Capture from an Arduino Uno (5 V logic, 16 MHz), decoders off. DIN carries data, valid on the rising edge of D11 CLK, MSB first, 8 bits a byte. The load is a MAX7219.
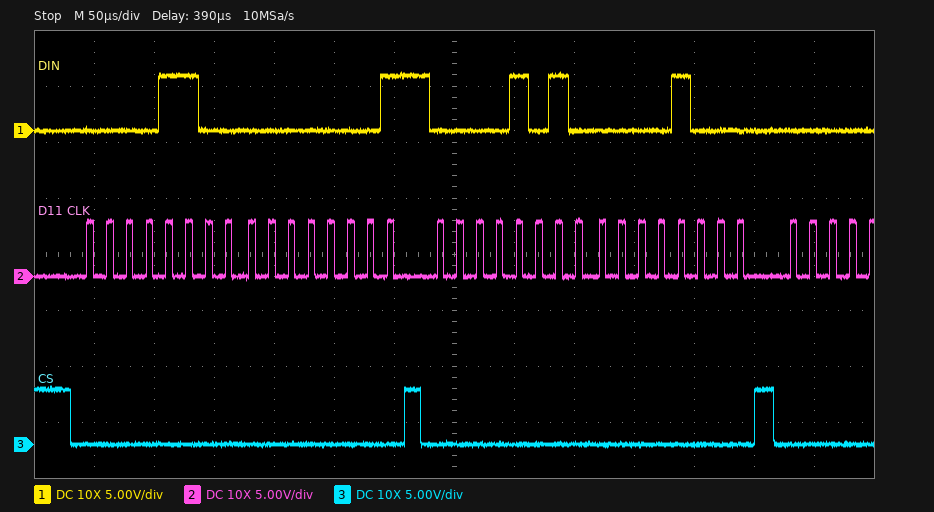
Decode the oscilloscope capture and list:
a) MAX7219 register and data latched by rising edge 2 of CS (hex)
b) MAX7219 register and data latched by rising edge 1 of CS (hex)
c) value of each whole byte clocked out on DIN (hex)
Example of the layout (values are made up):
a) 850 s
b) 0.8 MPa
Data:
a) register 0xA, data 0x08
b) register 0xC, data 0x01
c) 0C 01 0A 08
